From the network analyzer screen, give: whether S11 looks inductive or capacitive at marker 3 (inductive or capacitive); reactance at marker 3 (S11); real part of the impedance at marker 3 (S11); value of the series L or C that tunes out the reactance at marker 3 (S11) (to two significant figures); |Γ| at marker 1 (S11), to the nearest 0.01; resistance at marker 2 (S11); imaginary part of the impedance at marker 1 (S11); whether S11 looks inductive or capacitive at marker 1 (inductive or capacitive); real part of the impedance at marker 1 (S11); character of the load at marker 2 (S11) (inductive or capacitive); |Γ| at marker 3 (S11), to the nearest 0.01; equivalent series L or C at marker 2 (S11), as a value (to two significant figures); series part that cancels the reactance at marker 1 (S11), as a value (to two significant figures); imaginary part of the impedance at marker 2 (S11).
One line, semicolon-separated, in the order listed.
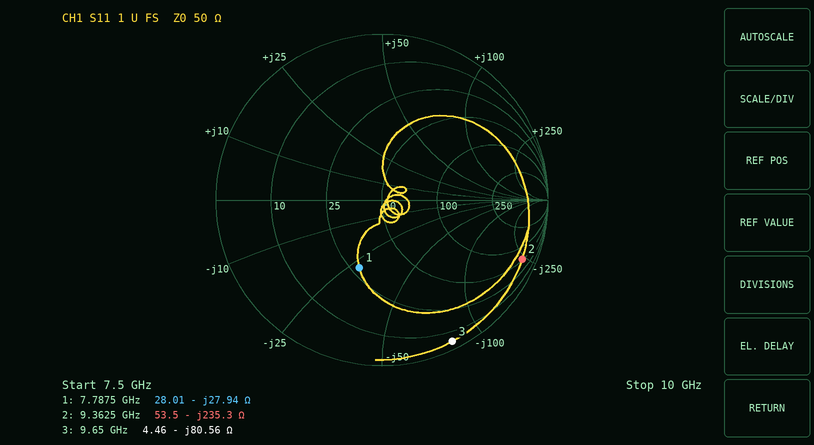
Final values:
capacitive; -80.56 Ω; 4.46 Ω; 1.3 nH; 0.43; 53.5 Ω; -27.94 Ω; capacitive; 28.01 Ω; capacitive; 0.95; 72 fF; 570 pH; -235.3 Ω
